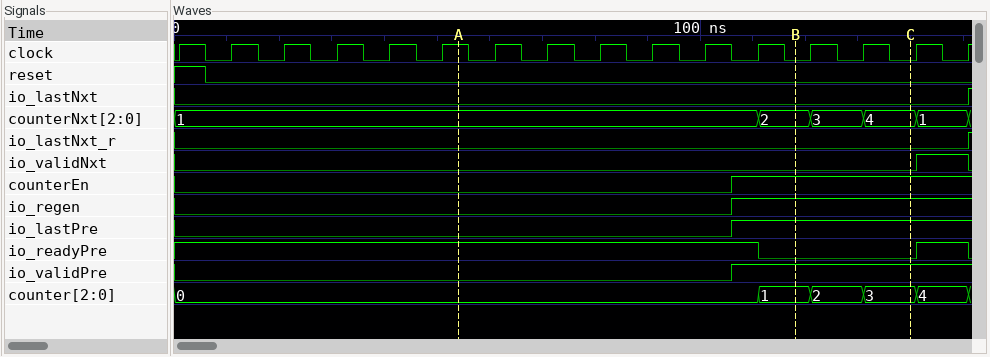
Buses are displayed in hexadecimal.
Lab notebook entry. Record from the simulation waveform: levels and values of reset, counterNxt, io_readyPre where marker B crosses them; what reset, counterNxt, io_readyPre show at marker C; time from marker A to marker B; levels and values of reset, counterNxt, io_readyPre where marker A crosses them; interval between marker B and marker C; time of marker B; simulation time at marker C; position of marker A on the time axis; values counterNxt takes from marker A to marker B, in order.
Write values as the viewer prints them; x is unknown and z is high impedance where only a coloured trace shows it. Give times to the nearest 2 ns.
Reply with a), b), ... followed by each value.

a) reset=0, counterNxt=2, io_readyPre=0
b) reset=0, counterNxt=4, io_readyPre=0
c) 64 ns
d) reset=0, counterNxt=1, io_readyPre=1
e) 22 ns
f) 118 ns
g) 140 ns
h) 54 ns
i) 1, 2
